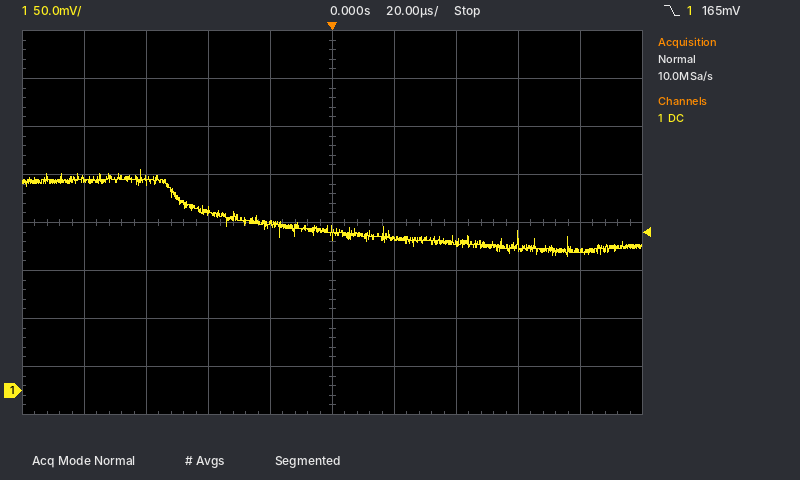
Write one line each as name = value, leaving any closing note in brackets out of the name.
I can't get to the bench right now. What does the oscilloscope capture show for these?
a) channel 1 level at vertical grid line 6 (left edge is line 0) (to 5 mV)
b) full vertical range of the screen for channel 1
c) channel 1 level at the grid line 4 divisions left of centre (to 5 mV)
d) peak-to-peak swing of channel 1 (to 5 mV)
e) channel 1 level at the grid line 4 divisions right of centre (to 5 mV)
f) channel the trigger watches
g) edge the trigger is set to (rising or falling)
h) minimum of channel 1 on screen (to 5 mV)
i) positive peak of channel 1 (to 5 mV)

channel 1 level at vertical grid line 6 (left edge is line 0) = 160 mV
full vertical range of the screen for channel 1 = 400 mV
channel 1 level at the grid line 4 divisions left of centre = 220 mV
peak-to-peak swing of channel 1 = 90 mV
channel 1 level at the grid line 4 divisions right of centre = 145 mV
channel the trigger watches = channel 1
edge the trigger is set to = falling
minimum of channel 1 on screen = 140 mV
positive peak of channel 1 = 230 mV
